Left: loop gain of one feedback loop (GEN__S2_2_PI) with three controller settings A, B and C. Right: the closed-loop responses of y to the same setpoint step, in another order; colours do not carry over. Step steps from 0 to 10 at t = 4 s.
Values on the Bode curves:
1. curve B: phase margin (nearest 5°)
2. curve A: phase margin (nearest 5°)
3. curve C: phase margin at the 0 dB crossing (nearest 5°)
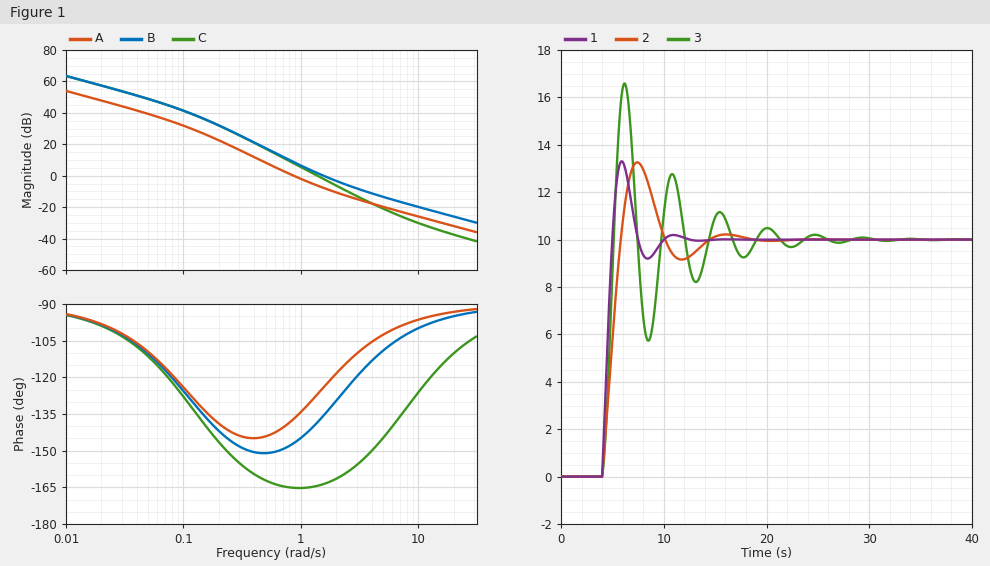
45°
45°
15°
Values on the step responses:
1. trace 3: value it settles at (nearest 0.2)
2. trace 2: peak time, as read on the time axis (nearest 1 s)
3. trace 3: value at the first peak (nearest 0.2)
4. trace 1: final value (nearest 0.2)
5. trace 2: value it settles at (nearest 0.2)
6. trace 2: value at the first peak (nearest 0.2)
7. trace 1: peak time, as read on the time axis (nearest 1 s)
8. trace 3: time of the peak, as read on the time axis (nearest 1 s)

10.0
7 s
16.6
10.0
10.0
13.2
6 s
6 s
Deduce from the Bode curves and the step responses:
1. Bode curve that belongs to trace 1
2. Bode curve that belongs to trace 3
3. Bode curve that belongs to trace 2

B
C
A
